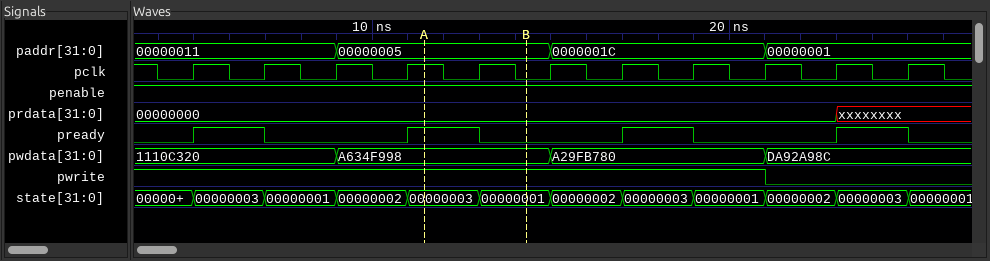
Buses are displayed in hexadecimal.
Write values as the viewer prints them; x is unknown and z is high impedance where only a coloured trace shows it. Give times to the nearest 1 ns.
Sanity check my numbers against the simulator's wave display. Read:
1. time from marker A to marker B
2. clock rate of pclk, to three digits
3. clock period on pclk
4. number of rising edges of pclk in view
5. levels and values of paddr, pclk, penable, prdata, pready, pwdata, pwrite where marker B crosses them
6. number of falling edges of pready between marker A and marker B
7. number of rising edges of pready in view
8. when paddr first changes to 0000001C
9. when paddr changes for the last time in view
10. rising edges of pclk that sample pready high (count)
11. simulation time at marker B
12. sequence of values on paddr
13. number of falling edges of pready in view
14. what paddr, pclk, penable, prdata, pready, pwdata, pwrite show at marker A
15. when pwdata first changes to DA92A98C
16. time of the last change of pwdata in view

3 ns
500 MHz
2 ns
11
paddr=00000005, pclk=0, penable=1, prdata=00000000, pready=0, pwdata=A634F998, pwrite=1
1
4
15 ns
21 ns
4
14 ns
00000011, 00000005, 0000001C, 00000001
4
paddr=00000005, pclk=1, penable=1, prdata=00000000, pready=1, pwdata=A634F998, pwrite=1
21 ns
21 ns
